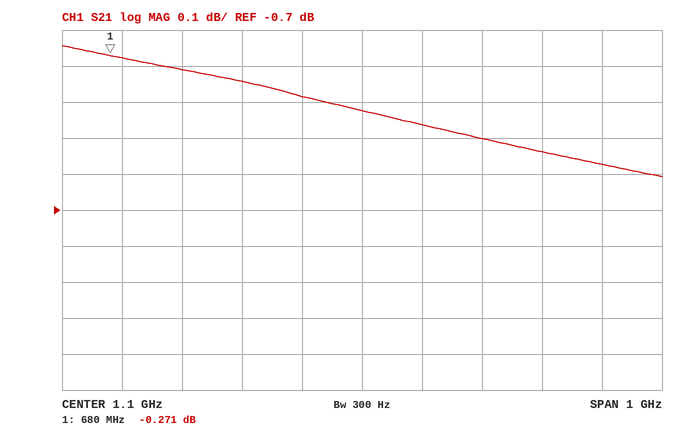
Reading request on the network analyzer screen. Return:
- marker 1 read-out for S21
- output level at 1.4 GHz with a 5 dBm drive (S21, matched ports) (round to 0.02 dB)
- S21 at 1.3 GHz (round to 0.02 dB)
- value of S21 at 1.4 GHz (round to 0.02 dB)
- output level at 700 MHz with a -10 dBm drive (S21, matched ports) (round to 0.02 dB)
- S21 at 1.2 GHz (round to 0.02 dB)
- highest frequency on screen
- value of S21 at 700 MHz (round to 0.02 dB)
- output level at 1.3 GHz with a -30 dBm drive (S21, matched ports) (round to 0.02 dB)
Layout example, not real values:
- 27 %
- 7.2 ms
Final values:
- -0.271 dB
- 4.46 dBm
- -0.50 dB
- -0.54 dB
- -10.28 dBm
- -0.46 dB
- 1.6 GHz
- -0.28 dB
- -30.50 dBm
